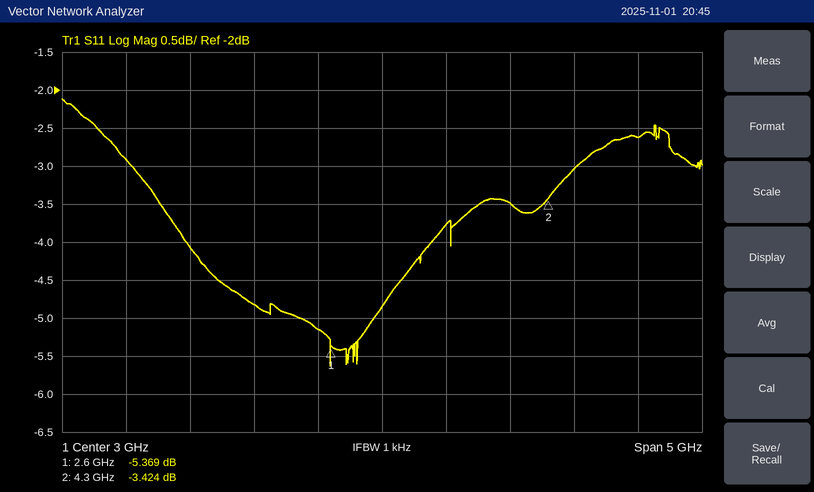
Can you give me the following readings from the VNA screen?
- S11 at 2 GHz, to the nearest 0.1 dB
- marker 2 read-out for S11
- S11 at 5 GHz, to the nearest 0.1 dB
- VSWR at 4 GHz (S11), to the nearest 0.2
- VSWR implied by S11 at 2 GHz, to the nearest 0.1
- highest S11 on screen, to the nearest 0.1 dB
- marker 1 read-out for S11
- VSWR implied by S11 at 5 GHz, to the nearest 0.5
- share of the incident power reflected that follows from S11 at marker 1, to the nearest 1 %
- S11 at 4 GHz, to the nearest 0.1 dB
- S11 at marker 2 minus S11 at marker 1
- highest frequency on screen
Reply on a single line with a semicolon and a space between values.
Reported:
-4.8 dB; -3.424 dB; -2.6 dB; 5.0; 3.7; -2.1 dB; -5.369 dB; 6.5; 29 %; -3.5 dB; 1.945 dB; 5.5 GHz
